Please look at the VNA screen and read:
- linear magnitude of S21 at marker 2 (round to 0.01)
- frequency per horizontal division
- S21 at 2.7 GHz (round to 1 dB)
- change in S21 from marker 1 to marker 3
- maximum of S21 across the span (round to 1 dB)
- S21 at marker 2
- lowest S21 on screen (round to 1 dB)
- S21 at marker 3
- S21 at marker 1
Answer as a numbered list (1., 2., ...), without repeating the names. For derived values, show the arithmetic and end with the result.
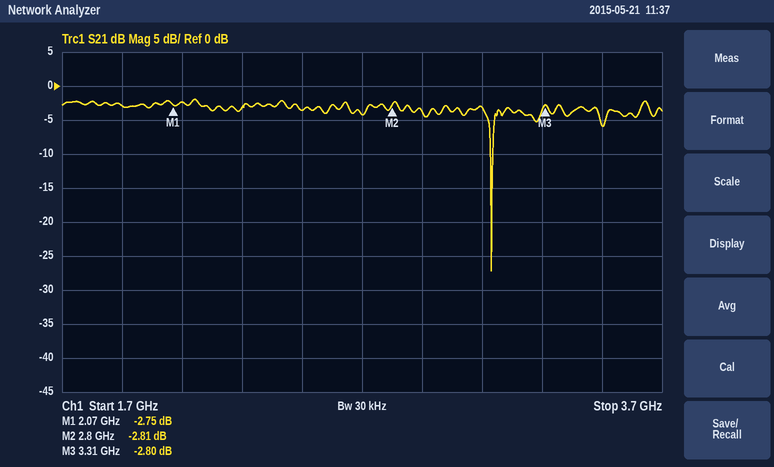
1. 10^(-2.81/20) ≈ 0.72
2. 200 MHz
3. -4 dB
4. -2.8 − (-2.75) = -0.05 dB
5. -2 dB
6. -2.81 dB
7. -27 dB
8. -2.80 dB
9. -2.75 dB
